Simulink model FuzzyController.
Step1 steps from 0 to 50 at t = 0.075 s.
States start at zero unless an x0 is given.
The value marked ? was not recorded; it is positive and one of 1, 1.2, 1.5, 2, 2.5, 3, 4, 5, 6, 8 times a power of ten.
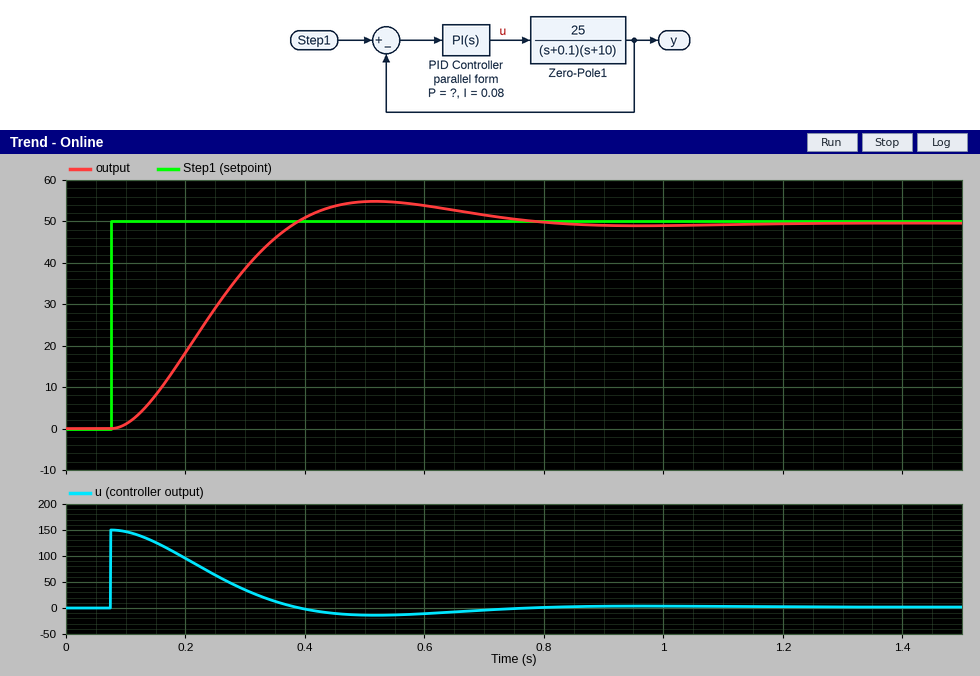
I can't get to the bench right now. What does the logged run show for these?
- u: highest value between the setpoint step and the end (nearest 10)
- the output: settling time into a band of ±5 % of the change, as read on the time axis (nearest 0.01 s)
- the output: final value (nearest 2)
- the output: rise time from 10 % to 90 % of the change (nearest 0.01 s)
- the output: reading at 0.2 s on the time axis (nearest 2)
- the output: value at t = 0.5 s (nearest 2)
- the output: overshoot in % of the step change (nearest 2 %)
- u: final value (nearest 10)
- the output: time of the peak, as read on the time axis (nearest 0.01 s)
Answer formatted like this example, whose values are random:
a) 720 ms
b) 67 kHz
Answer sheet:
a) 150
b) 0.68 s
c) 50
d) 0.21 s
e) 18
f) 54
g) 10 %
h) 0
i) 0.52 s
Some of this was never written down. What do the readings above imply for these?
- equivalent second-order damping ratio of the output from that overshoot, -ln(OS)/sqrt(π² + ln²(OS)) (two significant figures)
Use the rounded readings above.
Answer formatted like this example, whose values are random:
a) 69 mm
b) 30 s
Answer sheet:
a) 0.59
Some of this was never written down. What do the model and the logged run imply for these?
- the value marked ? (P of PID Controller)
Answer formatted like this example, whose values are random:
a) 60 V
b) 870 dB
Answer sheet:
a) 3
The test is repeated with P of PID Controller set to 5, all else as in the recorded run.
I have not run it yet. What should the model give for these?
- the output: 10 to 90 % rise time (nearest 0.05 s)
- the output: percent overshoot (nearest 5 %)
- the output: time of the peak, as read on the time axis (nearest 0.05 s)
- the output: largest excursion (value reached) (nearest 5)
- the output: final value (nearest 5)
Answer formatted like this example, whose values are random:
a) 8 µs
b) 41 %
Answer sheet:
a) 0.15 s
b) 20 %
c) 0.40 s
d) 60
e) 50
